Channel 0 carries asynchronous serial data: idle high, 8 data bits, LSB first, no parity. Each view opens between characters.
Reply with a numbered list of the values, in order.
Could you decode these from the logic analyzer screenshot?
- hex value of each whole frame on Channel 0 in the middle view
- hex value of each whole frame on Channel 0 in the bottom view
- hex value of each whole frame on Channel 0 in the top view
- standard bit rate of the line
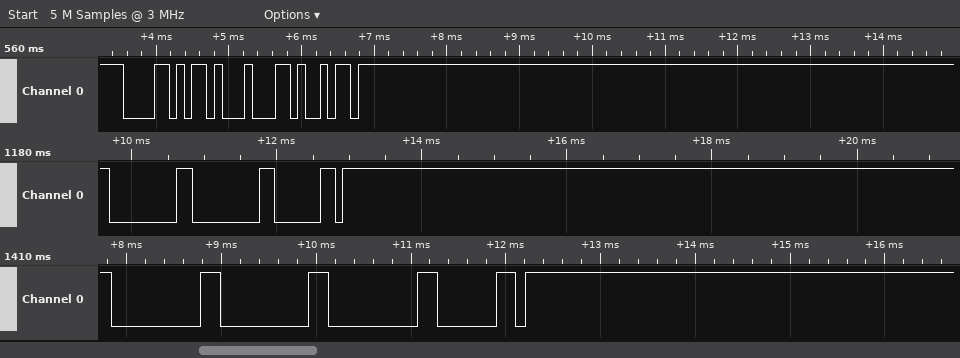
1. 00, 00, 60
2. 00, 00, 00, 60
3. 58, 11, 69
4. 9600 baud
